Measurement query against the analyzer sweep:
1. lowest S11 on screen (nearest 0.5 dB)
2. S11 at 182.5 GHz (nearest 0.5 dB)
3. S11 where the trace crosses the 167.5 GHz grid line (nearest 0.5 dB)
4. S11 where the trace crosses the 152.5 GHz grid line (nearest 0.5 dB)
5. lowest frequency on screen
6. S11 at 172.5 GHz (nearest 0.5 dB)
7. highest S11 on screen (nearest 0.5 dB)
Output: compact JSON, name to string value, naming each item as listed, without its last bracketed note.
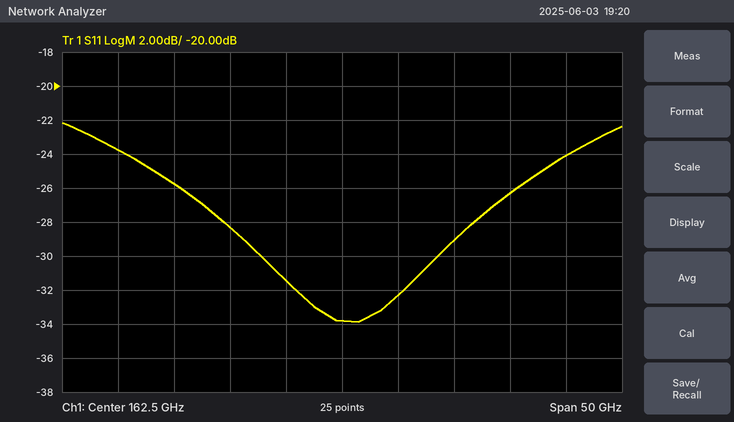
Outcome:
{"lowest S11 on screen": "-34.0 dB", "S11 at 182.5 GHz": "-24.0 dB", "S11 where the trace crosses the 167.5 GHz grid line": "-32.5 dB", "S11 where the trace crosses the 152.5 GHz grid line": "-28.5 dB", "lowest frequency on screen": "137.5 GHz", "S11 at 172.5 GHz": "-29.0 dB", "highest S11 on screen": "-22.0 dB"}
